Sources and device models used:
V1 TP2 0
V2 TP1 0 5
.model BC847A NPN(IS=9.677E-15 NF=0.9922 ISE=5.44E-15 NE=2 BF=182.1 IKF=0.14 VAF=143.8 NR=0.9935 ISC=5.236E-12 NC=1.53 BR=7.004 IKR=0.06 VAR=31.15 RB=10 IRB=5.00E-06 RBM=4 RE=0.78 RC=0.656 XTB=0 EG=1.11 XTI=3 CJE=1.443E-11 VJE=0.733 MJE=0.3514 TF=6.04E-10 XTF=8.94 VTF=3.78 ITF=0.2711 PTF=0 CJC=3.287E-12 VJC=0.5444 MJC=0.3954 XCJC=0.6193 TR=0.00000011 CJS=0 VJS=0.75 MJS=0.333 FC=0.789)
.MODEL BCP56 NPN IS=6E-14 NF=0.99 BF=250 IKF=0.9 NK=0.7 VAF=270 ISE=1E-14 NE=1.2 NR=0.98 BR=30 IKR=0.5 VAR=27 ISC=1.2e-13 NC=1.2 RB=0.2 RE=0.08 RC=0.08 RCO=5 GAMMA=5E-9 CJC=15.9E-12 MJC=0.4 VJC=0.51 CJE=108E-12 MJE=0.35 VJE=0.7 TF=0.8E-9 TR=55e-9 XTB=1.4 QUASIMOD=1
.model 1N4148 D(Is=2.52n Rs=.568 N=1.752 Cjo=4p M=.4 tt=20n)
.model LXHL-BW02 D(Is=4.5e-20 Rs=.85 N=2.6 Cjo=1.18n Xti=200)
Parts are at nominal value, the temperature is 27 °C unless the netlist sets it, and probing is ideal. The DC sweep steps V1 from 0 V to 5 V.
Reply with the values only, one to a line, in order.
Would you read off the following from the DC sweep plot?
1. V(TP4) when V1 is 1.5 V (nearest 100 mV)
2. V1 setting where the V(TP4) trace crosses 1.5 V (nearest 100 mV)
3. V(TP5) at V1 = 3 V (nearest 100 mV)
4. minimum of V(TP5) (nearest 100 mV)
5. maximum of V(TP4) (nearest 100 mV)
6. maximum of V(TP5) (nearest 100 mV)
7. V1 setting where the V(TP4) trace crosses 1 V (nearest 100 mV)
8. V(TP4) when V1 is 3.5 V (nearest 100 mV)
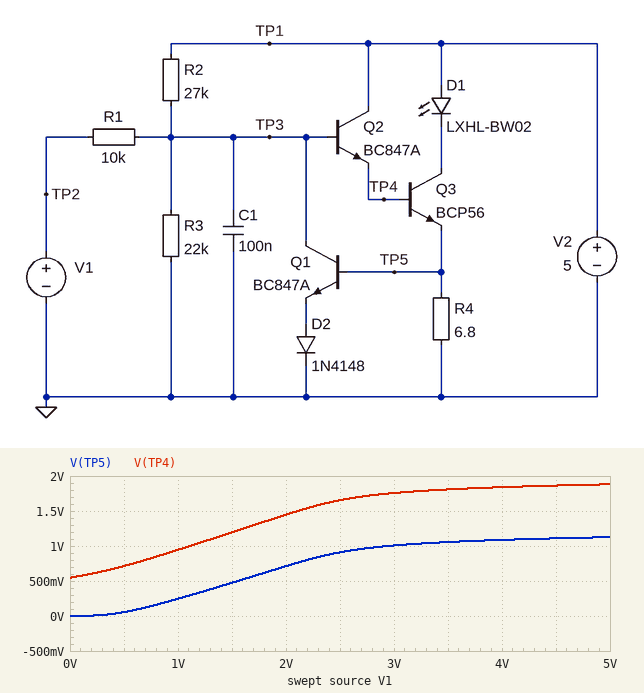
1.2 V
2.1 V
1.0 V
0 V
1.9 V
1.1 V
1.1 V
1.8 V
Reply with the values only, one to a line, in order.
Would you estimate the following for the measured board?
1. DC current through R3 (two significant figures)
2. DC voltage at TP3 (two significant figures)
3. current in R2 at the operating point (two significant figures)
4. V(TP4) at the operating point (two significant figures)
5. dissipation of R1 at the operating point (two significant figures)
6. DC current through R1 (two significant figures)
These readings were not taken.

46 µA
1.0 V
150 µA
550 mV
100 µW
100 µA
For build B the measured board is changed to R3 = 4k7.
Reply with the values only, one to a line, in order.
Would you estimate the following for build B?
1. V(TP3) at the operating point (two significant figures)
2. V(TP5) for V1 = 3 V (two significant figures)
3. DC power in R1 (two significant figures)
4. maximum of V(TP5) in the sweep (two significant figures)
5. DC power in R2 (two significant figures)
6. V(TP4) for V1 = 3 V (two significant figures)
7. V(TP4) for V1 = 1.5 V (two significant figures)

530 mV
120 mV
28 µW
590 mV
740 µW
790 mV
520 mV
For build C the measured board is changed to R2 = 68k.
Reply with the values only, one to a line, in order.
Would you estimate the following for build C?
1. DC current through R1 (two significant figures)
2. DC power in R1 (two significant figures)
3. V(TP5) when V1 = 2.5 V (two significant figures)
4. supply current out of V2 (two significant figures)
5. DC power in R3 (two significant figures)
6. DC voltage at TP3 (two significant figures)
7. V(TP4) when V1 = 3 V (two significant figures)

46 µA
21 µW
630 mV
67 µA
9.6 µW
460 mV
1.6 V
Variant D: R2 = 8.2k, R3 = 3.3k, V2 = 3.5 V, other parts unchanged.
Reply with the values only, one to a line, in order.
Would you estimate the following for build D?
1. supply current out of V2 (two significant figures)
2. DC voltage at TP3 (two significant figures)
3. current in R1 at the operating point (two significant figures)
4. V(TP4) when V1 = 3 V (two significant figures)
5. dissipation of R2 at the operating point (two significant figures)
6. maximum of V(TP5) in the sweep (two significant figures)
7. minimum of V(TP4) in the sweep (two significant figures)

330 µA
810 mV
81 µA
790 mV
880 µW
410 mV
440 mV
